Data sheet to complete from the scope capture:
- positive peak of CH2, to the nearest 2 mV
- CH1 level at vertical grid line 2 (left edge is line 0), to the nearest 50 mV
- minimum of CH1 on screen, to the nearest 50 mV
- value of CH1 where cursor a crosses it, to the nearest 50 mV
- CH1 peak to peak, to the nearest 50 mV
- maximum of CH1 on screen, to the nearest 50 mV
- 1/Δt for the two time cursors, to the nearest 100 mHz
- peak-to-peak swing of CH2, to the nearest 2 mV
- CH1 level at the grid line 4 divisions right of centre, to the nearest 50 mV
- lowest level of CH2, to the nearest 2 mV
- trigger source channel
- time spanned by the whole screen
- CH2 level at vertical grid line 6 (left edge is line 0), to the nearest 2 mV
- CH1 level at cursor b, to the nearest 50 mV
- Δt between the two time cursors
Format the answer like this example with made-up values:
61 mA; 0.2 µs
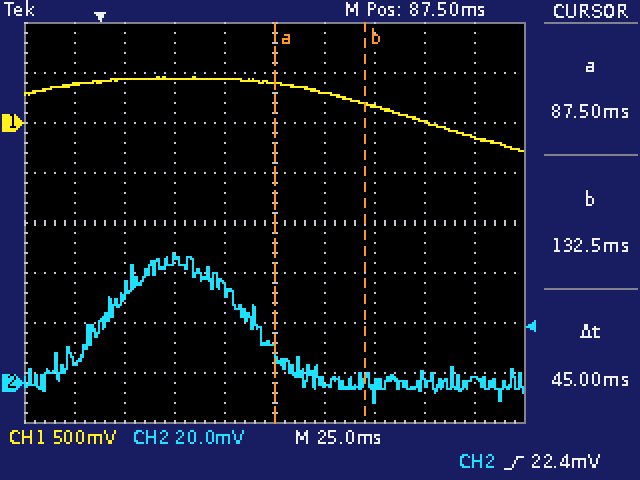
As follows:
52 mV; 450 mV; -300 mV; 400 mV; 750 mV; 450 mV; 22.2 Hz; 60 mV; -150 mV; -8 mV; CH2; 250 ms; 0 mV; 200 mV; 45 ms
